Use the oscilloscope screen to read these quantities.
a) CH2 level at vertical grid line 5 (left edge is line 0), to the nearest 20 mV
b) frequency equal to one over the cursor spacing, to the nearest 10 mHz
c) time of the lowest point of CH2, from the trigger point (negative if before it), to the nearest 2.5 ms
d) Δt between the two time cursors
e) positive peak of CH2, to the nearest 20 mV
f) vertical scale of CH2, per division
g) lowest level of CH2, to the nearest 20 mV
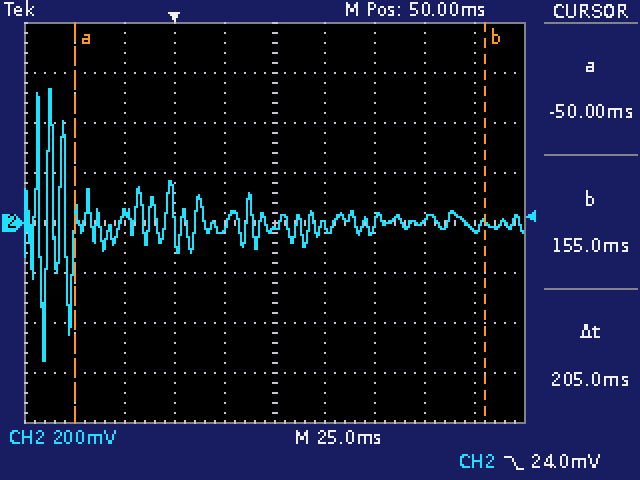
-20 mV
4.88 Hz
-65.0 ms
205 ms
540 mV
200 mV
-560 mV
